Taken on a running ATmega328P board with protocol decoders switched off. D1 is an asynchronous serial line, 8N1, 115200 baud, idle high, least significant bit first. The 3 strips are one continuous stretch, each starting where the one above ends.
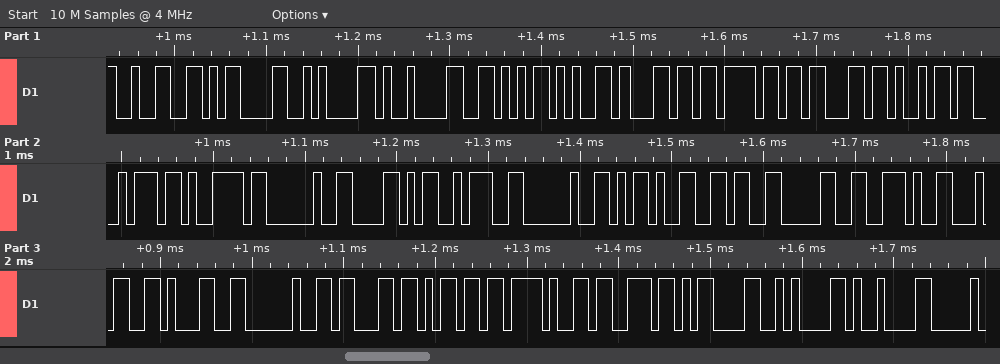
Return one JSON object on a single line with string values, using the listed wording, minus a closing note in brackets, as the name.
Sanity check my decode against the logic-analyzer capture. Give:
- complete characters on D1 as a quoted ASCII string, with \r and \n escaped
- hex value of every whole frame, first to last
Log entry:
{"complete characters on D1 as a quoted ASCII string, with \\r and \\n escaped": "\"2\\r\\n\\tVelocity X: -60.41 cm/s\\r\\n\\t\"", "hex value of every whole frame, first to last": "32 0D 0A 09 56 65 6C 6F 63 69 74 79 20 58 3A 20 2D 36 30 2E 34 31 20 63 6D 2F 73 0D 0A 09"}
